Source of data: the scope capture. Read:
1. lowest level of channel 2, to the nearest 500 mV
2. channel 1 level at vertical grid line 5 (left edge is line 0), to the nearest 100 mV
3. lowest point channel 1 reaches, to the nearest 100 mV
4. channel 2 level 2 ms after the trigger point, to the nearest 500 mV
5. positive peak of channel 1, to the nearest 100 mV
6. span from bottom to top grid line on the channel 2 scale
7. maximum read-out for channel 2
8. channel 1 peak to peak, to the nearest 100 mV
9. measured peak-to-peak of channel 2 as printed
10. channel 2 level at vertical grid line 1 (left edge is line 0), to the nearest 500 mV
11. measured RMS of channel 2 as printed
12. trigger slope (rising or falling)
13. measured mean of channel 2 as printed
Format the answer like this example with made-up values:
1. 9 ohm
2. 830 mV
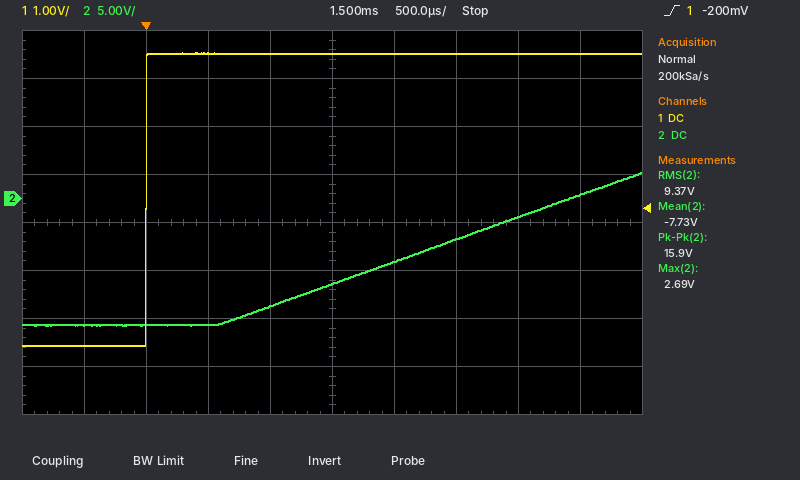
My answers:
1. -13.0 V
2. 3.0 V
3. -3.1 V
4. -6.5 V
5. 3.0 V
6. 40 V
7. 2.69 V
8. 6.1 V
9. 15.9 V
10. -13.0 V
11. 9.37 V
12. rising
13. -7.73 V
